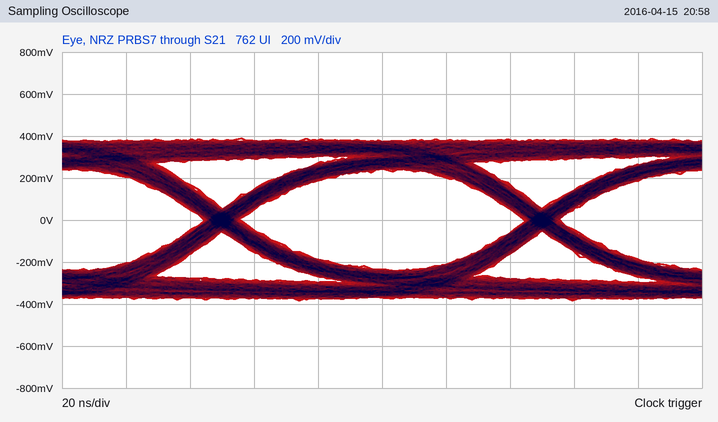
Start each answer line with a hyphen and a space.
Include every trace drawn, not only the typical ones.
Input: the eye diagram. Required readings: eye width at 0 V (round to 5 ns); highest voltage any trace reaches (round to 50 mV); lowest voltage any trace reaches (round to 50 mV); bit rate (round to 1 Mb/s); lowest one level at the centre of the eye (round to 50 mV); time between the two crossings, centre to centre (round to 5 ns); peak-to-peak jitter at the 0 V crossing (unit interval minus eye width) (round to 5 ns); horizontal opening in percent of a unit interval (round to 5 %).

- 90 ns
- 400 mV
- -400 mV
- 10 Mb/s
- 250 mV
- 100 ns
- 10 ns
- 90 %
